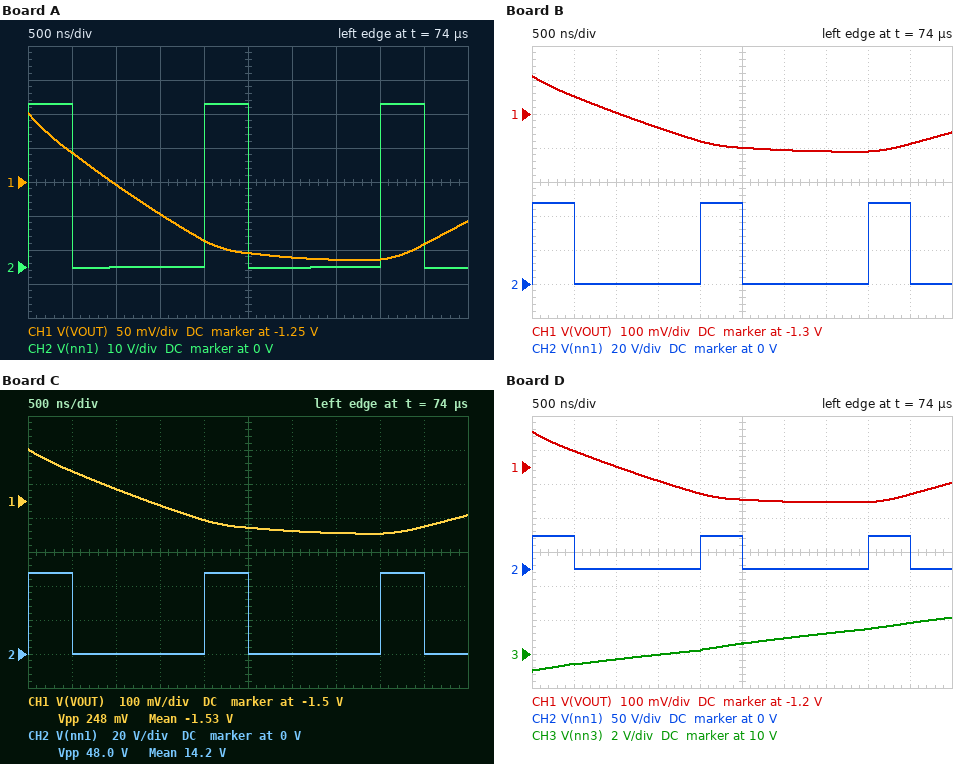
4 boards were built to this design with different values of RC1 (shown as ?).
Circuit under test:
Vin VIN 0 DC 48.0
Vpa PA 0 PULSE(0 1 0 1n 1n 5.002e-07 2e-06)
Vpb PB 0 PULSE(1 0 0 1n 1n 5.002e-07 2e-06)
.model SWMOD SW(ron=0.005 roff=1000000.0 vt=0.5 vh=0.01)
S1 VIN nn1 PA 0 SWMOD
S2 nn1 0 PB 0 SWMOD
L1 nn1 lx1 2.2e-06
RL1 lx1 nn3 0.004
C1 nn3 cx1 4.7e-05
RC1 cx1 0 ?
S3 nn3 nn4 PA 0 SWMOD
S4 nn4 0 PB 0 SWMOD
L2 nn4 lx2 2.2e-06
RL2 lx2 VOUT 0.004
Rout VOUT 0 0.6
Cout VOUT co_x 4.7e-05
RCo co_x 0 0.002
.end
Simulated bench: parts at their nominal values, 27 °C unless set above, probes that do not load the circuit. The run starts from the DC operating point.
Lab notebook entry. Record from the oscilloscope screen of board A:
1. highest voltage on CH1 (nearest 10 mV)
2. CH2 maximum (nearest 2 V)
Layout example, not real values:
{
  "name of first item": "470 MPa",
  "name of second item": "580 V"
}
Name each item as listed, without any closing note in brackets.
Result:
{
  "highest voltage on CH1": "-1.15 V",
  "CH2 maximum": "48 V"
}
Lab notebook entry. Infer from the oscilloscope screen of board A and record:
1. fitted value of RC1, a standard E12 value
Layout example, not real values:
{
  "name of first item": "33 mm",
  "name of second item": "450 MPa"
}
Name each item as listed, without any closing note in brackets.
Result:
{
  "fitted value of RC1, a standard E12 value": "5.6 mΩ"
}
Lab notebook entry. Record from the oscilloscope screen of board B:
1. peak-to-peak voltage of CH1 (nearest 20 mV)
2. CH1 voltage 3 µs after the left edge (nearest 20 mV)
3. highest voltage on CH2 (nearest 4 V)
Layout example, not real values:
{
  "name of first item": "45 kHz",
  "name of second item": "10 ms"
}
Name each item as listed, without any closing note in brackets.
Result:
{
  "peak-to-peak voltage of CH1": "220 mV",
  "CH1 voltage 3 µs after the left edge": "-1.40 V",
  "highest voltage on CH2": "48 V"
}
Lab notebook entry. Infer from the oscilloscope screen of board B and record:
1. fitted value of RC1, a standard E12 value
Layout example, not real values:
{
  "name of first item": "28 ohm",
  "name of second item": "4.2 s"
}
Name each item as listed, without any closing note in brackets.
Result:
{
  "fitted value of RC1, a standard E12 value": "4.7 mΩ"
}
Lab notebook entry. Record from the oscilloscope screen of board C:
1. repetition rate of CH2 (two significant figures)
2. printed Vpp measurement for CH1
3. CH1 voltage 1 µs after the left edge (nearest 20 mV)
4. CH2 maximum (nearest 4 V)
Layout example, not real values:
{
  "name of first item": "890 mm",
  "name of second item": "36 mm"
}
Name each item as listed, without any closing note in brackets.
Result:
{
  "repetition rate of CH2": "500 kHz",
  "printed Vpp measurement for CH1": "248 mV",
  "CH1 voltage 1 µs after the left edge": "-1.46 V",
  "CH2 maximum": "48 V"
}
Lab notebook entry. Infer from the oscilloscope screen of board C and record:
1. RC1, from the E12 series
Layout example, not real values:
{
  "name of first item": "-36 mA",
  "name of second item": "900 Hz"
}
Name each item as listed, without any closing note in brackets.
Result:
{
  "RC1, from the E12 series": "1.2 mΩ"
}
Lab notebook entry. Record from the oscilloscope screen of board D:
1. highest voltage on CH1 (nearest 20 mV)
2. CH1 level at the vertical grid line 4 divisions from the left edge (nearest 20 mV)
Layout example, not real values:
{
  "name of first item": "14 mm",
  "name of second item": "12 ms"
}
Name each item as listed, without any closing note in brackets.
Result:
{
  "highest voltage on CH1": "-1.10 V",
  "CH1 level at the vertical grid line 4 divisions from the left edge": "-1.28 V"
}
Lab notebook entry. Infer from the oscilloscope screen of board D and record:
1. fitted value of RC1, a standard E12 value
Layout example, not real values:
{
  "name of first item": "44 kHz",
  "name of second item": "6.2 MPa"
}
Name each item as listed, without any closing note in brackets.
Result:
{
  "fitted value of RC1, a standard E12 value": "6.8 mΩ"
}
